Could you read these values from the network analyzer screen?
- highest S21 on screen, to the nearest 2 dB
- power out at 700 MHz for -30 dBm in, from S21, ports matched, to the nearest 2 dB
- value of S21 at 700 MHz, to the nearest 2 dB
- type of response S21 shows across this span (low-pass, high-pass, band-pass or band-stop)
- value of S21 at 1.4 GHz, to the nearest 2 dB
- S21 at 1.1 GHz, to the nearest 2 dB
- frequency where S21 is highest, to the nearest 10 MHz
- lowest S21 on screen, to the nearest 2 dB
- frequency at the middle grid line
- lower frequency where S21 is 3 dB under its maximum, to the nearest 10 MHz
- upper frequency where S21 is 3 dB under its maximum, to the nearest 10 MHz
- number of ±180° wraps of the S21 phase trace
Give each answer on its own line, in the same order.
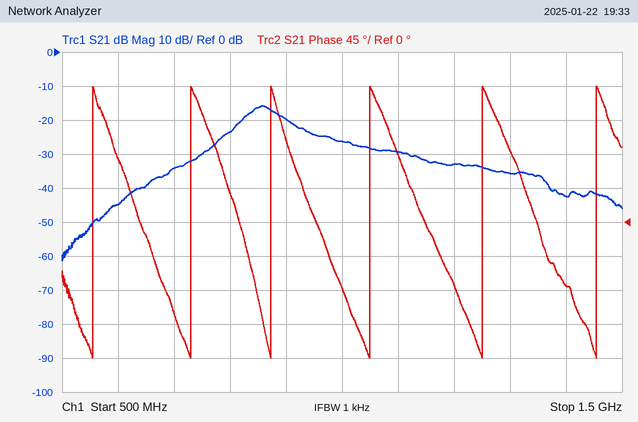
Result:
-16 dB
-64 dBm
-34 dB
band-pass
-42 dB
-30 dB
860 MHz
-62 dB
1 GHz
830 MHz
890 MHz
6
